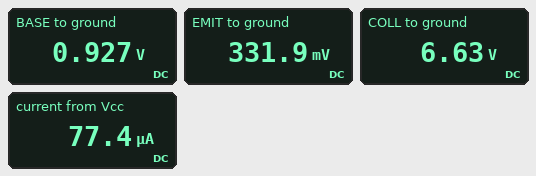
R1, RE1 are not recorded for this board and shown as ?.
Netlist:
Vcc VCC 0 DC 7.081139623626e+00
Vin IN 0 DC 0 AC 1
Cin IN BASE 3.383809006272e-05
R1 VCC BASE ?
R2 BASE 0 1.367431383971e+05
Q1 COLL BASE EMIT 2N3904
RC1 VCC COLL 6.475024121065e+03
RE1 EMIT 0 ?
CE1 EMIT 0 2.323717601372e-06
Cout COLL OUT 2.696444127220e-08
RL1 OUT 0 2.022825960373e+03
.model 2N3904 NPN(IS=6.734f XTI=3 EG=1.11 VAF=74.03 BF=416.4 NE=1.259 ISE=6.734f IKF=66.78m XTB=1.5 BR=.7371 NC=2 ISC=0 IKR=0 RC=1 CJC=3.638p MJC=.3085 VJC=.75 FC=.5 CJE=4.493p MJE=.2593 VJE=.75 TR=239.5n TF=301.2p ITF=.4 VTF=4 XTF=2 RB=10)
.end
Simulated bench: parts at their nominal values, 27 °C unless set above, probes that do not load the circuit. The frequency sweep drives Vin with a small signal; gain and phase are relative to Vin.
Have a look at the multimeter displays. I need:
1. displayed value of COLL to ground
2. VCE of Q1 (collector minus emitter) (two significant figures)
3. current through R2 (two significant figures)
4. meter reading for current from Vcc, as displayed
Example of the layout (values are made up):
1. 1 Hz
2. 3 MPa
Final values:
1. 6.63 V
2. 6.3 V
3. 6.8 µA
4. 77.4 µA
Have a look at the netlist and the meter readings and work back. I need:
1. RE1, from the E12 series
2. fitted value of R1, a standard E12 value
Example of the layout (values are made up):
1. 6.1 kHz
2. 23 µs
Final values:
1. 4.7 kΩ
2. 820 kΩ
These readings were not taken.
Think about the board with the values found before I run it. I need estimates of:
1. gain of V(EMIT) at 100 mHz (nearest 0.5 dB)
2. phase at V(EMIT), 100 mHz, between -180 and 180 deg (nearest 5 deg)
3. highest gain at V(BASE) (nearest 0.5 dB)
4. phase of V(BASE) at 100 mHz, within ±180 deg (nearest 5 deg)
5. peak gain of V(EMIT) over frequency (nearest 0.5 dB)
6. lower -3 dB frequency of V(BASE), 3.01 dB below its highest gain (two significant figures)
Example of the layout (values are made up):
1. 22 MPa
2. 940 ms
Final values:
1. -1.5 dB
2. 25 deg
3. 0 dB
4. 25 deg
5. -0.5 dB
6. 48 mHz
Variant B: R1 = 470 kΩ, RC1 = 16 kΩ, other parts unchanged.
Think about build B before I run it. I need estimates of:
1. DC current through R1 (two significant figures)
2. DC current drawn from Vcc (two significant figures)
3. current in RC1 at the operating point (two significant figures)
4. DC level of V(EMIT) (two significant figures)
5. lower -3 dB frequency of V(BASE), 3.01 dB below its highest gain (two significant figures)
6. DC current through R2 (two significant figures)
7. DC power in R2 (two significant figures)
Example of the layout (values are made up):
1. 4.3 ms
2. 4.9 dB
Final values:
1. 12 µA
2. 180 µA
3. 170 µA
4. 810 mV
5. 52 mHz
6. 10 µA
7. 15 µW
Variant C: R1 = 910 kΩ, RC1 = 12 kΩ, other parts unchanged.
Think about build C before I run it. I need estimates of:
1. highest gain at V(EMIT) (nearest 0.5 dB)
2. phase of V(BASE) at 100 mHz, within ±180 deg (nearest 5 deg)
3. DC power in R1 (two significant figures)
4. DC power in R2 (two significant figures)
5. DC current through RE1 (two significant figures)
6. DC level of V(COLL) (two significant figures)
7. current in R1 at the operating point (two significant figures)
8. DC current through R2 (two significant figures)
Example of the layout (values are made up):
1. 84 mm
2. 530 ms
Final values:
1. -1.0 dB
2. 25 deg
3. 43 µW
4. 5.3 µW
5. 56 µA
6. 6.4 V
7. 6.8 µA
8. 6.2 µA
